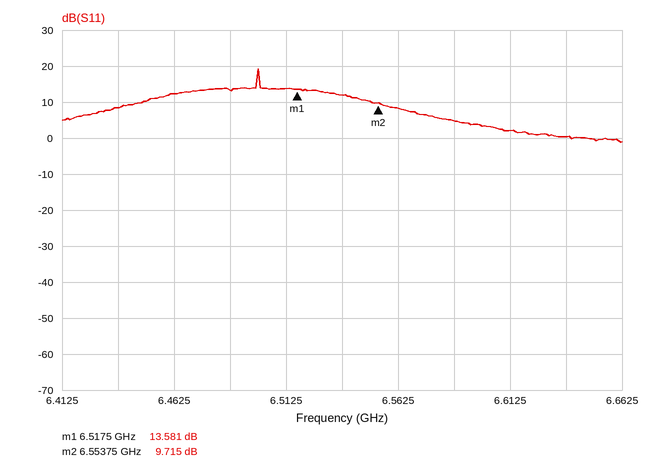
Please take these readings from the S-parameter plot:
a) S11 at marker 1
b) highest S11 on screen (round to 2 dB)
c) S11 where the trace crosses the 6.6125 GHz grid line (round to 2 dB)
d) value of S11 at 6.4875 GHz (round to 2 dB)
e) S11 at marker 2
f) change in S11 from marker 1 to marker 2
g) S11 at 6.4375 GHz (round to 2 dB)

13.581 dB
20 dB
2 dB
14 dB
9.715 dB
-3.866 dB
8 dB
